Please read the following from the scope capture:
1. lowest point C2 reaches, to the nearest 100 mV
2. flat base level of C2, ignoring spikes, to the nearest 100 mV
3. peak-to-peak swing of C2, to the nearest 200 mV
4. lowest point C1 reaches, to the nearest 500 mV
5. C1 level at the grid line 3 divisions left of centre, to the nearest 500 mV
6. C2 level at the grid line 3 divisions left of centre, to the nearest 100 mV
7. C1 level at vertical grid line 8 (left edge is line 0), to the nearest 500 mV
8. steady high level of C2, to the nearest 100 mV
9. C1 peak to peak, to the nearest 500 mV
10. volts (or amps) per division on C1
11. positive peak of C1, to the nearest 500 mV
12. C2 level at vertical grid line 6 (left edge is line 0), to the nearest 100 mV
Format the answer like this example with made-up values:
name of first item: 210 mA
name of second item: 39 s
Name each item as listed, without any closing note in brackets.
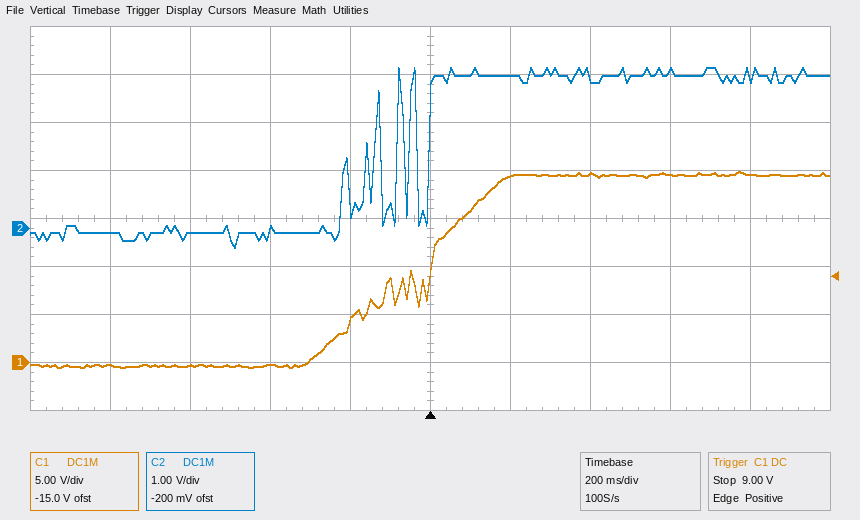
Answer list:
lowest point C2 reaches, to the nearest 100 mV: -400 mV
flat base level of C2, ignoring spikes, to the nearest 100 mV: -100 mV
peak-to-peak swing of C2, to the nearest 200 mV: 3.8 V
lowest point C1 reaches, to the nearest 500 mV: -500 mV
C1 level at the grid line 3 divisions left of centre, to the nearest 500 mV: -500 mV
C2 level at the grid line 3 divisions left of centre, to the nearest 100 mV: -100 mV
C1 level at vertical grid line 8 (left edge is line 0), to the nearest 500 mV: 19.5 V
steady high level of C2, to the nearest 100 mV: 3.2 V
C1 peak to peak, to the nearest 500 mV: 20.5 V
volts (or amps) per division on C1: 5 V
positive peak of C1, to the nearest 500 mV: 20.0 V
C2 level at vertical grid line 6 (left edge is line 0), to the nearest 100 mV: 3.2 V
